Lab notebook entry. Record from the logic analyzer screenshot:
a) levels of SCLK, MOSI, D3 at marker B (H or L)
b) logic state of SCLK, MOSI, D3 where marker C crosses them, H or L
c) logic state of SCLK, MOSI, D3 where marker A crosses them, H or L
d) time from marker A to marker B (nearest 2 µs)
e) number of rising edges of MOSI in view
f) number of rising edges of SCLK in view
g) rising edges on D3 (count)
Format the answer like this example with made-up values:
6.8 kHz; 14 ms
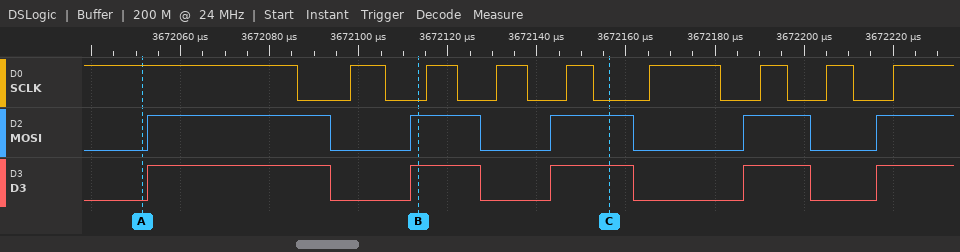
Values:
SCLK=L, MOSI=H, D3=H; SCLK=L, MOSI=H, D3=H; SCLK=H, MOSI=L, D3=L; 62 µs; 5; 8; 5
